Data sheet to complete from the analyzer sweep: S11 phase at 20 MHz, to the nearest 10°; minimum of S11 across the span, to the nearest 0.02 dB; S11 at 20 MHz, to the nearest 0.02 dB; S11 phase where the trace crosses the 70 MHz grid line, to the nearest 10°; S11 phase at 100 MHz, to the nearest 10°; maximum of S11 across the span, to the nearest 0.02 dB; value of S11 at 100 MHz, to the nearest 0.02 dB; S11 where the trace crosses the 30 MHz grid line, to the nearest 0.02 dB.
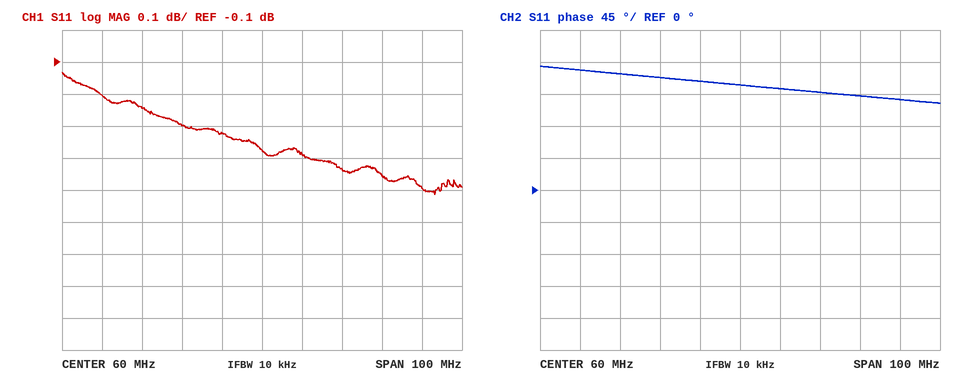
170°
-0.52 dB
-0.20 dB
140°
130°
-0.14 dB
-0.50 dB
-0.24 dB
